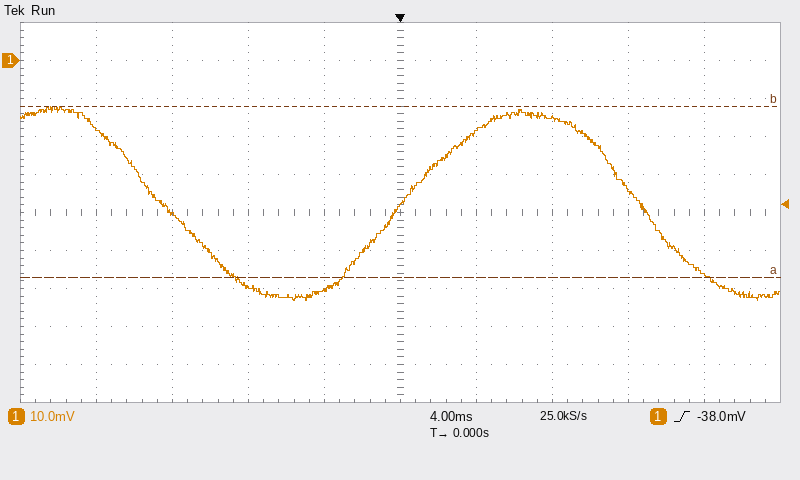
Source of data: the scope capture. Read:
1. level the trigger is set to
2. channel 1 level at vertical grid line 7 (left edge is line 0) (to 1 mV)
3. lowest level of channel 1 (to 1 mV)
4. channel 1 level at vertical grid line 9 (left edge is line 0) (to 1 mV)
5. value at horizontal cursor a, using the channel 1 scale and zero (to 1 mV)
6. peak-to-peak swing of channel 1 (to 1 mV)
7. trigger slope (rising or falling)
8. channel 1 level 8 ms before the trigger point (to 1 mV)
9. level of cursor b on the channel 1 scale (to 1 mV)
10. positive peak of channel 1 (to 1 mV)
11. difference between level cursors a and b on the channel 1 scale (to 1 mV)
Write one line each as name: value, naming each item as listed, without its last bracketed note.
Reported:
level the trigger is set to: -38.0 mV
channel 1 level at vertical grid line 7 (left edge is line 0): -15 mV
lowest level of channel 1: -63 mV
channel 1 level at vertical grid line 9 (left edge is line 0): -56 mV
value at horizontal cursor a, using the channel 1 scale and zero: -57 mV
peak-to-peak swing of channel 1: 51 mV
trigger slope: rising
channel 1 level 8 ms before the trigger point: -59 mV
level of cursor b on the channel 1 scale: -12 mV
positive peak of channel 1: -12 mV
difference between level cursors a and b on the channel 1 scale: 45 mV
